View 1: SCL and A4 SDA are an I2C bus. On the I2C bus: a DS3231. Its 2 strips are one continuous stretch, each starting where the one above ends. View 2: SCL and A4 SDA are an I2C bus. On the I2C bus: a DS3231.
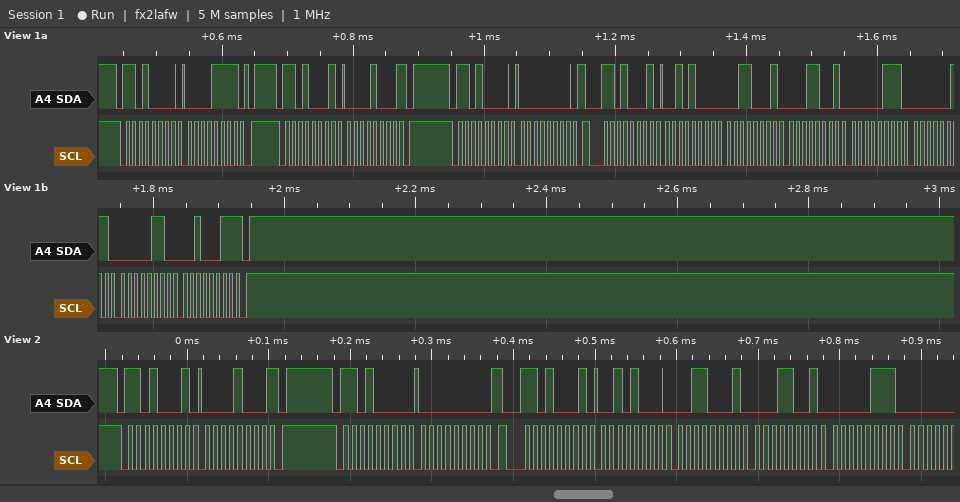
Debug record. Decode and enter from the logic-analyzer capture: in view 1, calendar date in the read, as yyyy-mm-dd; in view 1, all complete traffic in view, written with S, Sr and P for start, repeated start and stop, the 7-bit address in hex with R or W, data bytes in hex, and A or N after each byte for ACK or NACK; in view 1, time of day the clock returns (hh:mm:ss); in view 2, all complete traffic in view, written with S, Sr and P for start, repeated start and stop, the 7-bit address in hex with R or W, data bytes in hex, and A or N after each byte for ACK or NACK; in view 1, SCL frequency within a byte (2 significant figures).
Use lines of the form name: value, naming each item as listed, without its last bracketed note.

in view 1, calendar date in the read, as yyyy-mm-dd: 2023-06-03
in view 1, all complete traffic in view, written with S, Sr and P for start, repeated start and stop, the 7-bit address in hex with R or W, data bytes in hex, and A or N after each byte for ACK or NACK: S 68W A 0F A P S 68R A 08 N P S 68W A 00 A Sr 68R A 28 A 31 A 19 A 07 A 03 A 06 A 23 N P
in view 1, time of day the clock returns: 19:31:28
in view 2, all complete traffic in view, written with S, Sr and P for start, repeated start and stop, the 7-bit address in hex with R or W, data bytes in hex, and A or N after each byte for ACK or NACK: S 68R A 08 N P S 68W A 00 A Sr 68R A 28 A 31 A 19 A 07 A
in view 1, SCL frequency within a byte: 100 kHz
